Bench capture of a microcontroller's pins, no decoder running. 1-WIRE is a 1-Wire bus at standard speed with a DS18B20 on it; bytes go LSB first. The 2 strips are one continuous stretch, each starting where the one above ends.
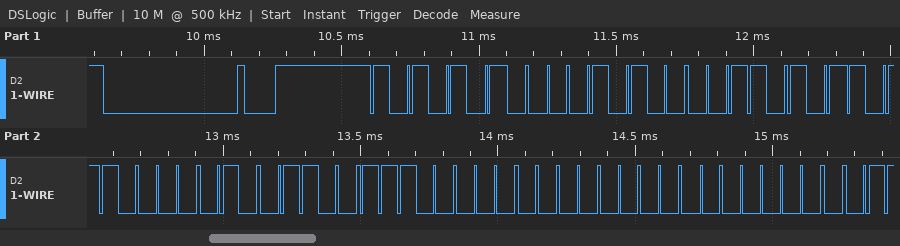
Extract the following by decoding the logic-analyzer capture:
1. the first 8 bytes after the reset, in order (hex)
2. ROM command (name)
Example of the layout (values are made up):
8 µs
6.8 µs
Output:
55 28 AC 0D 32 07 00 00
Match ROM
